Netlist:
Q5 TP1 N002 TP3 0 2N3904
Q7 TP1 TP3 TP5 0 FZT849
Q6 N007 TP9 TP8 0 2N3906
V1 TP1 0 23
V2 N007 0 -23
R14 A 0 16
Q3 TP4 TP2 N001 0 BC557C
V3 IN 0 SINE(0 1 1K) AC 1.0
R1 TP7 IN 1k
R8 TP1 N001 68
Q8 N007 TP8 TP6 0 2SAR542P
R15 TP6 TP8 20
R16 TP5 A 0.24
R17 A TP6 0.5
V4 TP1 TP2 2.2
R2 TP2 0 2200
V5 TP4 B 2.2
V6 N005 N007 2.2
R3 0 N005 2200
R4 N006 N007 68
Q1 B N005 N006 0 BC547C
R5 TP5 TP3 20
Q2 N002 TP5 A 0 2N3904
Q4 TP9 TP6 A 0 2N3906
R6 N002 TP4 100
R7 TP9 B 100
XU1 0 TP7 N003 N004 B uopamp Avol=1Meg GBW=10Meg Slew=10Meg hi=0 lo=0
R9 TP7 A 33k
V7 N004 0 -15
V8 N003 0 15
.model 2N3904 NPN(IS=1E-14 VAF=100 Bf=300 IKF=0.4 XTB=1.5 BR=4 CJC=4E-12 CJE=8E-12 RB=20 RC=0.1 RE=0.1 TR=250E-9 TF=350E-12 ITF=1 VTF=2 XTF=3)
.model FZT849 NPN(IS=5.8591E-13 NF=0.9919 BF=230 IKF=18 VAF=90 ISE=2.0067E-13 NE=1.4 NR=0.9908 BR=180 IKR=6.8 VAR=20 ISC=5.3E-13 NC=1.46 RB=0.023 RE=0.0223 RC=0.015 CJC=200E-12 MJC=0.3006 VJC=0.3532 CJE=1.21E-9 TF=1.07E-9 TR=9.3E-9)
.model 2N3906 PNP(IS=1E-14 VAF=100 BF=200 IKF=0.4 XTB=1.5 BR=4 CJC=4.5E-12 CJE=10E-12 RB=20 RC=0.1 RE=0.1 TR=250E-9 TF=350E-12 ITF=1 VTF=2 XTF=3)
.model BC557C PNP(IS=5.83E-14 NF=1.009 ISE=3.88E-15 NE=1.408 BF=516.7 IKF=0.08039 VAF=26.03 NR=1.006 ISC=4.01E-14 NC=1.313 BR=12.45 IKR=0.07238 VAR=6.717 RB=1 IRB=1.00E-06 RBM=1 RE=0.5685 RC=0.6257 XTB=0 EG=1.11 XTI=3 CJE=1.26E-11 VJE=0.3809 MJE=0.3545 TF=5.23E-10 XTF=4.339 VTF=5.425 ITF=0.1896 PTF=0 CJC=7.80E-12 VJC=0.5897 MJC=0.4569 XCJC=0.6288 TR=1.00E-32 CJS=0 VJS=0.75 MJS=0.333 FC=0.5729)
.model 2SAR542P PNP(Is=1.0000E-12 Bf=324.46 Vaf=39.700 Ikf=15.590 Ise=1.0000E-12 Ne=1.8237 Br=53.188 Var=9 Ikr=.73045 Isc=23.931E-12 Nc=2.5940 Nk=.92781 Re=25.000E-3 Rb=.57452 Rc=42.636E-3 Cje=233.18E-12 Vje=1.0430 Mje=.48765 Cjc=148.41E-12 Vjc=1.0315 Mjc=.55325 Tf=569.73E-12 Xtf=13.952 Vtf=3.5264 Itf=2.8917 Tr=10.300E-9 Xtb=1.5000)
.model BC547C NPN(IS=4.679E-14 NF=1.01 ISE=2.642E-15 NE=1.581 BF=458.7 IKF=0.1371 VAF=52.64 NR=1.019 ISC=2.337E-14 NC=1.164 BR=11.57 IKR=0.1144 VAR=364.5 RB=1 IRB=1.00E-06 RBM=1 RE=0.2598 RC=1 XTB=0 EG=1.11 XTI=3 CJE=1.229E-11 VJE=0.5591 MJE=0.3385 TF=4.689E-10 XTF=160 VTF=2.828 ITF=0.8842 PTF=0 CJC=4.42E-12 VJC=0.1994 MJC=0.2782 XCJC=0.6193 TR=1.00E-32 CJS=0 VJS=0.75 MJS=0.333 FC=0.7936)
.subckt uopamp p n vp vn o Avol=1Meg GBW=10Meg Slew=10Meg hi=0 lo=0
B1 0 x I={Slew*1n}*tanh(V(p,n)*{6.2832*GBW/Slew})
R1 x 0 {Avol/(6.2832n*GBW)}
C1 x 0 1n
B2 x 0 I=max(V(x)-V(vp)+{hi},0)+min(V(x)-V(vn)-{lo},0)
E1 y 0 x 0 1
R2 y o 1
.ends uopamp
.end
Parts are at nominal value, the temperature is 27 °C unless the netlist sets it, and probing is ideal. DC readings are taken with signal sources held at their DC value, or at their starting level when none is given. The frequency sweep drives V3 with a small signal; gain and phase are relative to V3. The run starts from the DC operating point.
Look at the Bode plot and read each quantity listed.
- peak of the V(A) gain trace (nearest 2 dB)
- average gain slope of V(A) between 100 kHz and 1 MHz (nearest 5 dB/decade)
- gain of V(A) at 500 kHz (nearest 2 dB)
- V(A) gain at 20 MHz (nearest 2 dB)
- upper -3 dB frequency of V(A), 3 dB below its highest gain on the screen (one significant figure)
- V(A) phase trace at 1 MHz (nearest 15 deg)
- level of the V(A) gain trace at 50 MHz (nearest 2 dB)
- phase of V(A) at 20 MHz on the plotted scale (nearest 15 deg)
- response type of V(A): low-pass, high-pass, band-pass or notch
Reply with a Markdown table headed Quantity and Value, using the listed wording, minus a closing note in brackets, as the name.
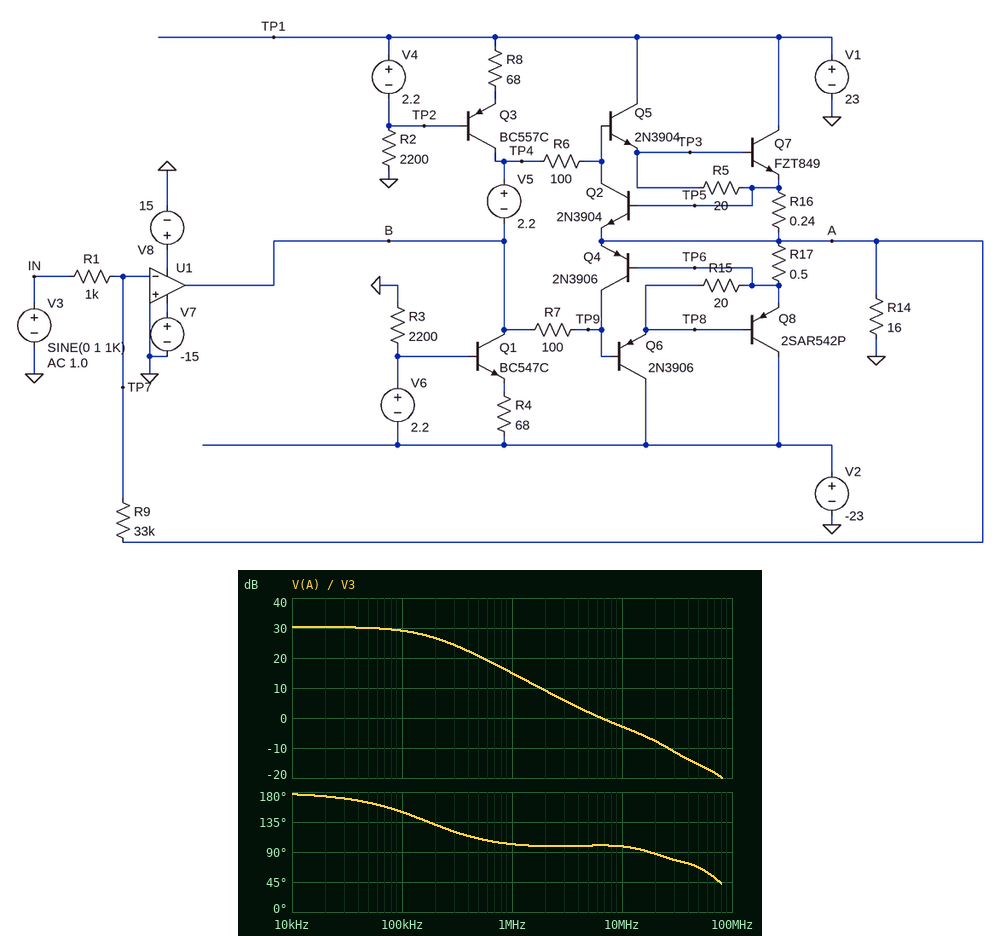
| Quantity | Value |
|---|---|
| peak of the V(A) gain trace | 30 dB |
| average gain slope of V(A) between 100 kHz and 1 MHz | -15 dB/decade |
| gain of V(A) at 500 kHz | 20 dB |
| V(A) gain at 20 MHz | -8 dB |
| upper -3 dB frequency of V(A), 3 dB below its highest gain on the screen | 200 kHz |
| V(A) phase trace at 1 MHz | 105 deg |
| level of the V(A) gain trace at 50 MHz | -16 dB |
| phase of V(A) at 20 MHz on the plotted scale | 90 deg |
| response type of V(A): low-pass, high-pass, band-pass or notch | low-pass |
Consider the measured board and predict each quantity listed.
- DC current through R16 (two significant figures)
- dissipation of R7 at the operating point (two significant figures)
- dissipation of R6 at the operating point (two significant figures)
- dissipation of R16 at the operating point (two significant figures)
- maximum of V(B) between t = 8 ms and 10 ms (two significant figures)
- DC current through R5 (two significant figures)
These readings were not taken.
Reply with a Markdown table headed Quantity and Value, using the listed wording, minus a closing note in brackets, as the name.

| Quantity | Value |
|---|---|
| DC current through R16 | 18 mA |
| dissipation of R7 at the operating point | 580 nW |
| dissipation of R6 at the operating point | 260 nW |
| dissipation of R16 at the operating point | 77 µW |
| maximum of V(B) between t = 8 ms and 10 ms | 15 V |
| DC current through R5 | 18 mA |
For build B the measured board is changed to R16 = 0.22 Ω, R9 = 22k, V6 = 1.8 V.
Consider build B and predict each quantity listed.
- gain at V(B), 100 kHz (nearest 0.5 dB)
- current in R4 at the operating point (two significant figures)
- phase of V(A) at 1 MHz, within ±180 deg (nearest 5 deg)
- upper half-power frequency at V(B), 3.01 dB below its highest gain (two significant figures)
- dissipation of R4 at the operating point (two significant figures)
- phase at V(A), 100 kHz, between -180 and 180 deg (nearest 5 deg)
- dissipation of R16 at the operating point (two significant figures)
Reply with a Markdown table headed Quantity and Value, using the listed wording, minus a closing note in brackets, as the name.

| Quantity | Value |
|---|---|
| gain at V(B), 100 kHz | 31.0 dB |
| current in R4 at the operating point | 16 mA |
| phase of V(A) at 1 MHz, within ±180 deg | 105 deg |
| upper half-power frequency at V(B), 3.01 dB below its highest gain | 250 kHz |
| dissipation of R4 at the operating point | 18 mW |
| phase at V(A), 100 kHz, between -180 and 180 deg | 160 deg |
| dissipation of R16 at the operating point | 71 µW |
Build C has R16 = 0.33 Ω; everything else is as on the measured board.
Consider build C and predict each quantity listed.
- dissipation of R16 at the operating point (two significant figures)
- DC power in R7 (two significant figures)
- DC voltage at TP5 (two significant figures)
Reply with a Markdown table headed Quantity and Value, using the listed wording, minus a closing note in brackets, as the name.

| Quantity | Value |
|---|---|
| dissipation of R16 at the operating point | 110 µW |
| DC power in R7 | 570 nW |
| DC voltage at TP5 | 5.9 mV |
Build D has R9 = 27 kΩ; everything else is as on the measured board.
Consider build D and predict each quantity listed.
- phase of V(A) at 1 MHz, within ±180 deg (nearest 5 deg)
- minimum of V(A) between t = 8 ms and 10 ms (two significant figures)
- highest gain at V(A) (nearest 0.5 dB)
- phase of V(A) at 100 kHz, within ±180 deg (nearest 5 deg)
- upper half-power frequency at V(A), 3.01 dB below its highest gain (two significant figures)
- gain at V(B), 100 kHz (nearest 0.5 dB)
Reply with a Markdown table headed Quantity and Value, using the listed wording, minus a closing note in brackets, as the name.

| Quantity | Value |
|---|---|
| phase of V(A) at 1 MHz, within ±180 deg | 105 deg |
| minimum of V(A) between t = 8 ms and 10 ms | -13 V |
| highest gain at V(A) | 28.5 dB |
| phase of V(A) at 100 kHz, within ±180 deg | 155 deg |
| upper half-power frequency at V(A), 3.01 dB below its highest gain | 210 kHz |
| gain at V(B), 100 kHz | 32.5 dB |
